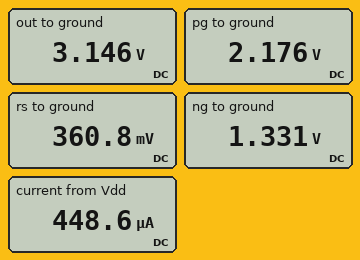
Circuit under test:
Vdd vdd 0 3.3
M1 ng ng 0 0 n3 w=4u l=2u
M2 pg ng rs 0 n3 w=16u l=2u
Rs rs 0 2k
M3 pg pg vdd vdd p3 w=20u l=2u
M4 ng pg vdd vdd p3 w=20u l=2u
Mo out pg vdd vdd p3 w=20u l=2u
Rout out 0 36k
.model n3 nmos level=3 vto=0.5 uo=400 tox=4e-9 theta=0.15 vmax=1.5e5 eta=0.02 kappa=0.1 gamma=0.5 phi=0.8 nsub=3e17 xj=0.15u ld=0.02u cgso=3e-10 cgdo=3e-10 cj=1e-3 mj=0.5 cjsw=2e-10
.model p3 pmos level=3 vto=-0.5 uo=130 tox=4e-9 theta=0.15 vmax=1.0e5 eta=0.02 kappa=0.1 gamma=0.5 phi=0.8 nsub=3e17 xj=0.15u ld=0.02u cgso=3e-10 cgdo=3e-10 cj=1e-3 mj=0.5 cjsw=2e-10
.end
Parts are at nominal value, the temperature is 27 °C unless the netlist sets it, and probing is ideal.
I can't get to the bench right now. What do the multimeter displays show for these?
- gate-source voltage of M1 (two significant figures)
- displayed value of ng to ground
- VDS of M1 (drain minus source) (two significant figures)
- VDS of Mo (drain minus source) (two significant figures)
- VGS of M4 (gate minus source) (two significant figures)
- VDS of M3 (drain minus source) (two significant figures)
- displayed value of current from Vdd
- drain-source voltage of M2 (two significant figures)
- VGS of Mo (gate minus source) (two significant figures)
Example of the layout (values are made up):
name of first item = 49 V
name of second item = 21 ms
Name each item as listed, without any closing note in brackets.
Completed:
gate-source voltage of M1 = 1.3 V
displayed value of ng to ground = 1.331 V
VDS of M1 (drain minus source) = 1.3 V
VDS of Mo (drain minus source) = -150 mV
VGS of M4 (gate minus source) = -1.1 V
VDS of M3 (drain minus source) = -1.1 V
displayed value of current from Vdd = 448.6 µA
drain-source voltage of M2 = 1.8 V
VGS of Mo (gate minus source) = -1.1 V
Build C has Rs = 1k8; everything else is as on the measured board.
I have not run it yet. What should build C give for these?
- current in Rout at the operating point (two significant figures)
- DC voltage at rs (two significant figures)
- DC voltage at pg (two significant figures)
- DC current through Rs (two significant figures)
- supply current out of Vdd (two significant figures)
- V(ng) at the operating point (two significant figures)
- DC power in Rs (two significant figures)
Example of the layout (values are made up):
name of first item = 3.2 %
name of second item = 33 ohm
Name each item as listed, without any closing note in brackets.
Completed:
current in Rout at the operating point = 88 µA
DC voltage at rs = 420 mV
DC voltage at pg = 2.1 V
DC current through Rs = 230 µA
supply current out of Vdd = 550 µA
V(ng) at the operating point = 1.5 V
DC power in Rs = 98 µW
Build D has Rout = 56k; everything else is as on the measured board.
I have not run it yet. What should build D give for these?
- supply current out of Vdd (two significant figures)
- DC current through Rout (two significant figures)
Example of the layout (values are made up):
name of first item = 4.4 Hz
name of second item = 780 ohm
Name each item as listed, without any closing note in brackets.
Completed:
supply current out of Vdd = 420 µA
DC current through Rout = 57 µA
